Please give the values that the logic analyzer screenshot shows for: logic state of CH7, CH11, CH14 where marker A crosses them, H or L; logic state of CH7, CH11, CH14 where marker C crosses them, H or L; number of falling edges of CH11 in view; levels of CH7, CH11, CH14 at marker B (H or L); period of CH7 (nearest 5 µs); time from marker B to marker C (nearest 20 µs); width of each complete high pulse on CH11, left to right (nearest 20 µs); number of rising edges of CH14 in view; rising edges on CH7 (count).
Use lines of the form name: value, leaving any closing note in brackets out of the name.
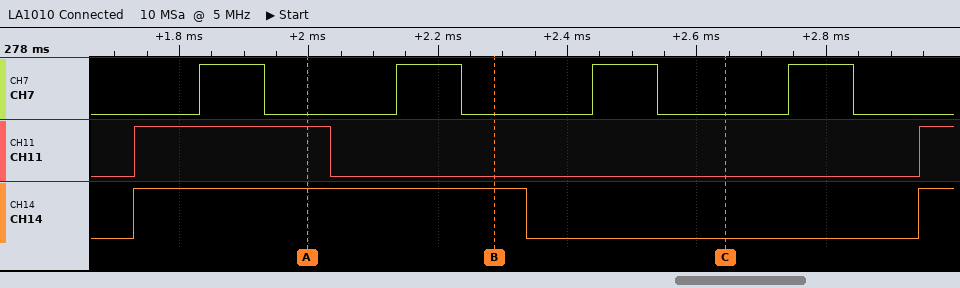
logic state of CH7, CH11, CH14 where marker A crosses them, H or L: CH7=L, CH11=H, CH14=H
logic state of CH7, CH11, CH14 where marker C crosses them, H or L: CH7=L, CH11=L, CH14=L
number of falling edges of CH11 in view: 1
levels of CH7, CH11, CH14 at marker B: CH7=L, CH11=L, CH14=H
period of CH7: 305 µs
time from marker B to marker C: 360 µs
width of each complete high pulse on CH11, left to right: 300 µs
number of rising edges of CH14 in view: 2
rising edges on CH7: 4
